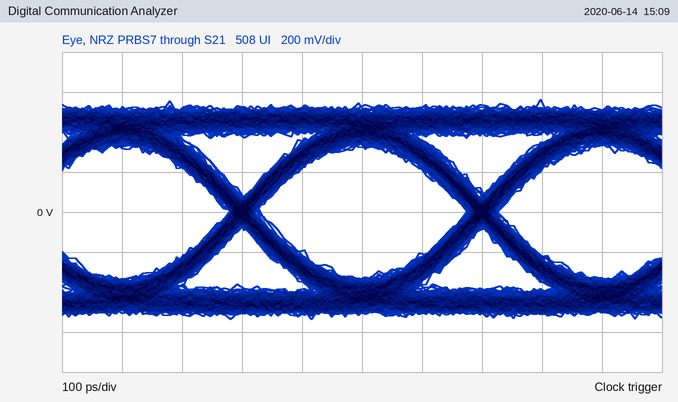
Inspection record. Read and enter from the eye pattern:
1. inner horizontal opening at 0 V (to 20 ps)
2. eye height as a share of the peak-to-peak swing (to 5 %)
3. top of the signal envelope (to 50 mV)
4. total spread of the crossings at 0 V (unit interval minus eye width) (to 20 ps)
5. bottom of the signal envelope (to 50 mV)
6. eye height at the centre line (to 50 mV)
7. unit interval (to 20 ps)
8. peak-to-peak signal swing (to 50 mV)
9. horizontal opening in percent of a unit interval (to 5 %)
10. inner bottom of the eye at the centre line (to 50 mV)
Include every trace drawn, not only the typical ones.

340 ps
60 %
550 mV
60 ps
-550 mV
650 mV
400 ps
1.10 V
85 %
-350 mV
